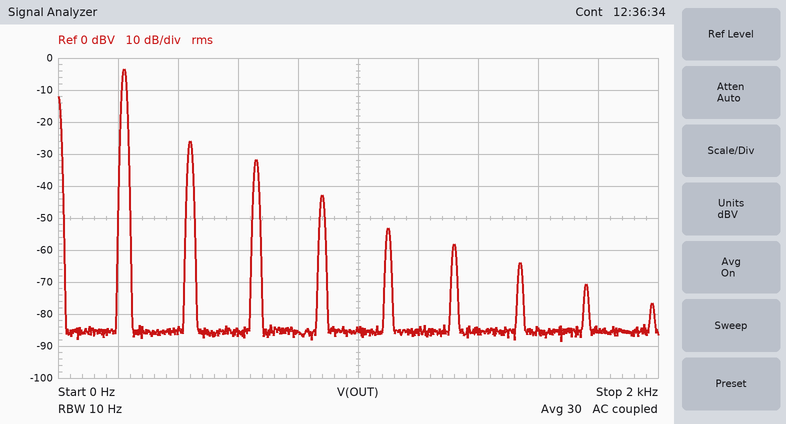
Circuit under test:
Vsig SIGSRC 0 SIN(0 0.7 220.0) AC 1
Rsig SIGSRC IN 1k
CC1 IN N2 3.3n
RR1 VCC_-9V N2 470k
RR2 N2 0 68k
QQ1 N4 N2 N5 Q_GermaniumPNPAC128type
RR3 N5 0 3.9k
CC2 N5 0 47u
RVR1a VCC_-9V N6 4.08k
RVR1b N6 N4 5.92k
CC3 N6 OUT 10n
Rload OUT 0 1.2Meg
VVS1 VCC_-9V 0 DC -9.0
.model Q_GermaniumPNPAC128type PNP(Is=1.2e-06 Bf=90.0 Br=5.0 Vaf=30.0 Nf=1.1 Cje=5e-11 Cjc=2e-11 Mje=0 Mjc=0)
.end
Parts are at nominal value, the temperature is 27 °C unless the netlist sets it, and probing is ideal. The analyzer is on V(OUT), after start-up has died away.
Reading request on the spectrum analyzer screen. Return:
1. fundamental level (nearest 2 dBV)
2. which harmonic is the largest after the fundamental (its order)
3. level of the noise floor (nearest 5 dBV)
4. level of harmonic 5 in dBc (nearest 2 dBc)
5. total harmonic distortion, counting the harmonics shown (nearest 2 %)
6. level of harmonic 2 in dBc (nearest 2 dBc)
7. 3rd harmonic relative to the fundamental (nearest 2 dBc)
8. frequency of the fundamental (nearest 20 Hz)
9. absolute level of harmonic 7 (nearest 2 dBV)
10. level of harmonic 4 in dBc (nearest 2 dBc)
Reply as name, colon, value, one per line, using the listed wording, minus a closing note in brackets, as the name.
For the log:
fundamental level: -4 dBV
which harmonic is the largest after the fundamental: 2
level of the noise floor: -85 dBV
level of harmonic 5 in dBc: -50 dBc
total harmonic distortion, counting the harmonics shown: 8 %
level of harmonic 2 in dBc: -22 dBc
3rd harmonic relative to the fundamental: -28 dBc
frequency of the fundamental: 220 Hz
absolute level of harmonic 7: -64 dBV
level of harmonic 4 in dBc: -40 dBc
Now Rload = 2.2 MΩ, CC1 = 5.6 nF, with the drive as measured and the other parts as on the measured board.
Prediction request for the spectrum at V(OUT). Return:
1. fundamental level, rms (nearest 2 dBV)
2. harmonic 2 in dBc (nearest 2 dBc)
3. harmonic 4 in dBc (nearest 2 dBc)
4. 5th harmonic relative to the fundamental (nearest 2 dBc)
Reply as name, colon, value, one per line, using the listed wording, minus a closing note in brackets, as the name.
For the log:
fundamental level, rms: 0 dBV
harmonic 2 in dBc: -12 dBc
harmonic 4 in dBc: -28 dBc
5th harmonic relative to the fundamental: -30 dBc
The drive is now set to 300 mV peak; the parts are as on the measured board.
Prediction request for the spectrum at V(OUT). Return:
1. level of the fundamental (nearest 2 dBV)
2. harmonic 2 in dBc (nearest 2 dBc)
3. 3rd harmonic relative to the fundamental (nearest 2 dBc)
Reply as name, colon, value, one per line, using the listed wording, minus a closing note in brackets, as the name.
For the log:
level of the fundamental: -10 dBV
harmonic 2 in dBc: -36 dBc
3rd harmonic relative to the fundamental: -46 dBc
